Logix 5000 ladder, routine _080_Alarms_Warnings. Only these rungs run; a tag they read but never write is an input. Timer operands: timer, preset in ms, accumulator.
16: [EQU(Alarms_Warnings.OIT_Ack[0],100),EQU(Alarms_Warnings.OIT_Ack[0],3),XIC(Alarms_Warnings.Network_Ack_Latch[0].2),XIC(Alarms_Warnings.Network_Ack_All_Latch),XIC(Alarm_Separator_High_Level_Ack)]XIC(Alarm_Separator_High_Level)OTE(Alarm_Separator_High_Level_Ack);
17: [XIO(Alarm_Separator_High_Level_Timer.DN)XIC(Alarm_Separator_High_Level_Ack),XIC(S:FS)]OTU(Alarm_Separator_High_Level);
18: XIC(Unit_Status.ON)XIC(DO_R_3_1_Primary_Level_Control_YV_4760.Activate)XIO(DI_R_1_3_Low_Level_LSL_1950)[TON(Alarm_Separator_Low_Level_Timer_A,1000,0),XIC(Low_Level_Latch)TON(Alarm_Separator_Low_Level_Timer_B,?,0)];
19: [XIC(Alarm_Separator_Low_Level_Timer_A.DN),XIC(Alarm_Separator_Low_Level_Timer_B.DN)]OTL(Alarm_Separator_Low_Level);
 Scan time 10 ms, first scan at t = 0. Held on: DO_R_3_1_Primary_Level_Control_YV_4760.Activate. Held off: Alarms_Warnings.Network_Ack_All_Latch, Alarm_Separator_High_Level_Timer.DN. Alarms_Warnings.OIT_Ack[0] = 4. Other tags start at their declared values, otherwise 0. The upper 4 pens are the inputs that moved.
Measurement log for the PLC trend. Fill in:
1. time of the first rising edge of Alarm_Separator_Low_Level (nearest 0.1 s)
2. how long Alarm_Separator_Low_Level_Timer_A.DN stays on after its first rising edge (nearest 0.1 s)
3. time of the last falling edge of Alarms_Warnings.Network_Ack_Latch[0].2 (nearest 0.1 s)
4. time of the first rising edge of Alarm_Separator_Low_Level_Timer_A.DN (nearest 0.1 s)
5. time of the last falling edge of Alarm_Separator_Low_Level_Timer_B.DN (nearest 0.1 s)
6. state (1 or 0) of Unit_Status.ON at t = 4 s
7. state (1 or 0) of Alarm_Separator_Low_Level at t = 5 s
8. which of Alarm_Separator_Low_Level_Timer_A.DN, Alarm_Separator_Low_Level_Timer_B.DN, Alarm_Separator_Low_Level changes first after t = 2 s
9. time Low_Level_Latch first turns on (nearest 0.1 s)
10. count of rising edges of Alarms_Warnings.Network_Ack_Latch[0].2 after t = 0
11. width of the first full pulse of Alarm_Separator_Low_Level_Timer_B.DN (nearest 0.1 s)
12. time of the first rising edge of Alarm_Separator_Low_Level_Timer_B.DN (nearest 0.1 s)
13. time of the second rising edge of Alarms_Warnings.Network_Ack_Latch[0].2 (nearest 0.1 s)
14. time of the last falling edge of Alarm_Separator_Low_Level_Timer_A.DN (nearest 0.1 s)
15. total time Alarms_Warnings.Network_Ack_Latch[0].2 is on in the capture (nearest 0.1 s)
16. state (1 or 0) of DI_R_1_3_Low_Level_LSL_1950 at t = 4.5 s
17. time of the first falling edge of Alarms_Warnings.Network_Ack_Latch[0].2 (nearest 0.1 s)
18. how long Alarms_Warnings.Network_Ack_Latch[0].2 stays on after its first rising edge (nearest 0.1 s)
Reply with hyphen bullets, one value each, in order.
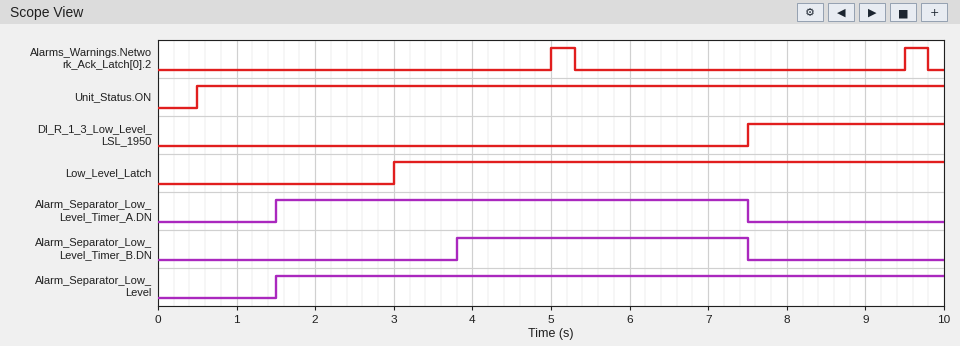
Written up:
- 1.5 s
- 6.0 s
- 9.8 s
- 1.5 s
- 7.5 s
- 1
- 1
- Alarm_Separator_Low_Level_Timer_B.DN
- 3.0 s
- 2
- 3.7 s
- 3.8 s
- 9.5 s
- 7.5 s
- 0.6 s
- 0
- 5.3 s
- 0.3 s
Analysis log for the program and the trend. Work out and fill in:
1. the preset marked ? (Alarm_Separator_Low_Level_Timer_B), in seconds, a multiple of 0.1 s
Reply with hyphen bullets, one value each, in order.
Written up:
- 0.8 s
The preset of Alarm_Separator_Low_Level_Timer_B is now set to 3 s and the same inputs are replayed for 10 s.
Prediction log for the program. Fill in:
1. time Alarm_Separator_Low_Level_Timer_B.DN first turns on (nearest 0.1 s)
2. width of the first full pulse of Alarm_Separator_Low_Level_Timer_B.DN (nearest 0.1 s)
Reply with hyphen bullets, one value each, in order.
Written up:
- 6.0 s
- 1.5 s
